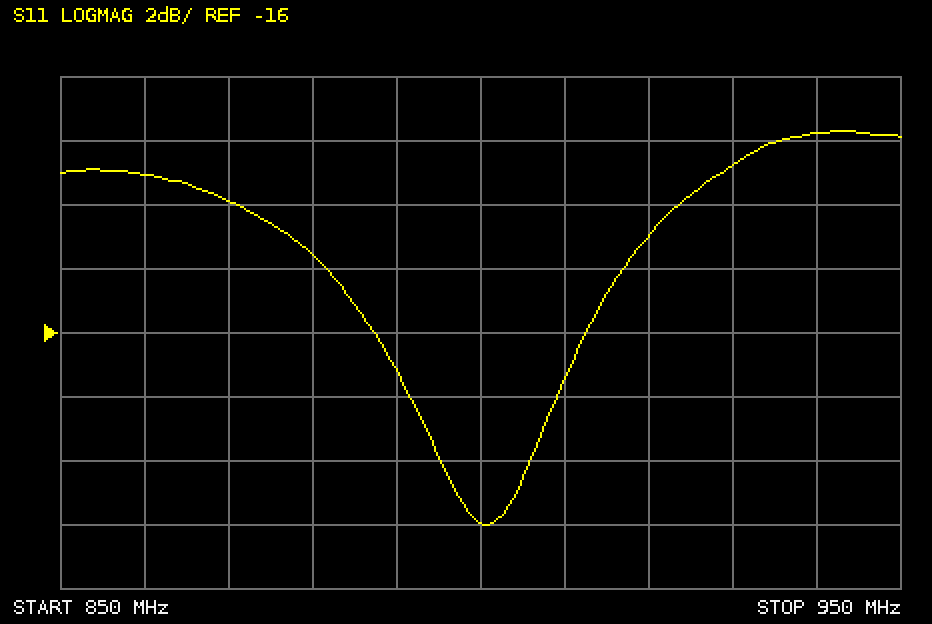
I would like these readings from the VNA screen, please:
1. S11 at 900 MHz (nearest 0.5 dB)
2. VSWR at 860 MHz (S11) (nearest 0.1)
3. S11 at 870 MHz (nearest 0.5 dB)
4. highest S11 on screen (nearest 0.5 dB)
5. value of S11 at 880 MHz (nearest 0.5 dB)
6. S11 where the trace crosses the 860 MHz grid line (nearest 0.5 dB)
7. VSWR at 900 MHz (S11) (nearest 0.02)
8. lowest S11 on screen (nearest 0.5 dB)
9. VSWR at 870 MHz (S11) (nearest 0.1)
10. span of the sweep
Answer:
-22.0 dB
1.8
-12.0 dB
-9.5 dB
-13.5 dB
-11.0 dB
1.18
-22.0 dB
1.7
100 MHz
